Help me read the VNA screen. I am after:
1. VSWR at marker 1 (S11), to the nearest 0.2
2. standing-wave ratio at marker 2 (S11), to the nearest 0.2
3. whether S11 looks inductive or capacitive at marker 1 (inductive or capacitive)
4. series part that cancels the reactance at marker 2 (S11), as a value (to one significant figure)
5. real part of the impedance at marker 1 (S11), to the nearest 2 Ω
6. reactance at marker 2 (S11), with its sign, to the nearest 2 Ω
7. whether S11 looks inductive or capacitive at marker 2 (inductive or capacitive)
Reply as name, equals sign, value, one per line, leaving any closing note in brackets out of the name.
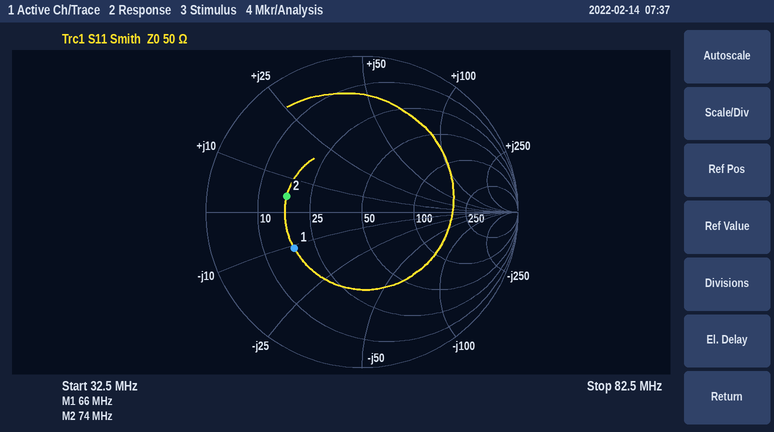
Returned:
VSWR at marker 1 (S11), to the nearest 0.2 = 3.0
standing-wave ratio at marker 2 (S11), to the nearest 0.2 = 3.0
whether S11 looks inductive or capacitive at marker 1 = capacitive
series part that cancels the reactance at marker 2 (S11), as a value = 500 pF
real part of the impedance at marker 1 (S11), to the nearest 2 Ω = 18 Ω
reactance at marker 2 (S11), with its sign, to the nearest 2 Ω = +4 Ω
whether S11 looks inductive or capacitive at marker 2 = inductive
